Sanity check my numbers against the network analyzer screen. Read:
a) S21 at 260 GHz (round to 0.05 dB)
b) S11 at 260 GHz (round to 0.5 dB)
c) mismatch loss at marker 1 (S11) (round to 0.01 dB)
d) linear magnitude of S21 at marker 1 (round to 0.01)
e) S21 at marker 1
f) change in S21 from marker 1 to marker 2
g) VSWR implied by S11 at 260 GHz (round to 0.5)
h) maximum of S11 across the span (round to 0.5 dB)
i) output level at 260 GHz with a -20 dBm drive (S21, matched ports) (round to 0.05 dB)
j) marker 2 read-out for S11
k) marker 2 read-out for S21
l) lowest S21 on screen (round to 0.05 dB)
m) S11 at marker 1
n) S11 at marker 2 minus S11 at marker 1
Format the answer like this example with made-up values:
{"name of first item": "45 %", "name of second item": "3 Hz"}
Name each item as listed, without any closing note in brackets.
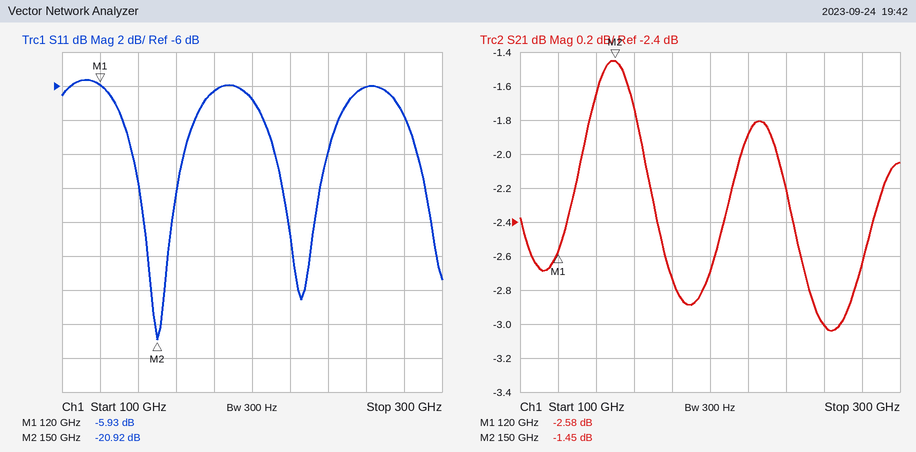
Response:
{"S21 at 260 GHz": "-3.00 dB", "S11 at 260 GHz": "-6.0 dB", "mismatch loss at marker 1 (S11)": "1.28 dB", "linear magnitude of S21 at marker 1": "0.74", "S21 at marker 1": "-2.58 dB", "change in S21 from marker 1 to marker 2": "1.13 dB", "VSWR implied by S11 at 260 GHz": "3.0", "maximum of S11 across the span": "-5.5 dB", "output level at 260 GHz with a -20 dBm drive (S21, matched ports)": "-23.00 dBm", "marker 2 read-out for S11": "-20.92 dB", "marker 2 read-out for S21": "-1.45 dB", "lowest S21 on screen": "-3.05 dB", "S11 at marker 1": "-5.93 dB", "S11 at marker 2 minus S11 at marker 1": "-14.99 dB"}
